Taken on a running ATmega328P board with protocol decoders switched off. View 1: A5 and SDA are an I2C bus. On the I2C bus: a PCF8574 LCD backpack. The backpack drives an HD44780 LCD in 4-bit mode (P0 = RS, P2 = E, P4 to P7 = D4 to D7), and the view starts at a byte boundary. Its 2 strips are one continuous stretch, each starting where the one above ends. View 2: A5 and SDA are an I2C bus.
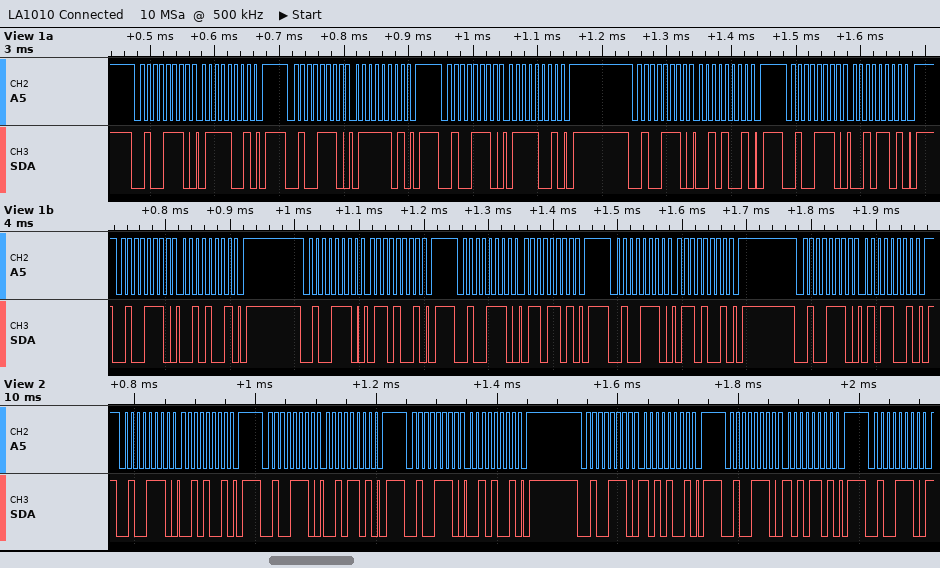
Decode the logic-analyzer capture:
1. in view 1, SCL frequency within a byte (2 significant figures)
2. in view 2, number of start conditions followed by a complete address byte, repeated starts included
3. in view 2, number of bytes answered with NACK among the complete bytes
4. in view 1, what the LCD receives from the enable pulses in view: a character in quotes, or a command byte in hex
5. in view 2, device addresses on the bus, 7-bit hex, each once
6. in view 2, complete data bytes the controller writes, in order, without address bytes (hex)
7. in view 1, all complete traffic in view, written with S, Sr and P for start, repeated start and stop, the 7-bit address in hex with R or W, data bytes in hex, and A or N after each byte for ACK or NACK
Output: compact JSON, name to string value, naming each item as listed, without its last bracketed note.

{"in view 1, SCL frequency within a byte": "100 kHz", "in view 2, number of start conditions followed by a complete address byte, repeated starts included": "6", "in view 2, number of bytes answered with NACK among the complete bytes": "0", "in view 1, what the LCD receives from the enable pulses in view: a character in quotes, or a command byte in hex": "'r'", "in view 2, device addresses on the bus, 7-bit hex, each once": "0x27", "in view 2, complete data bytes the controller writes, in order, without address bytes": "29 2D 29 A9 AD", "in view 1, all complete traffic in view, written with S, Sr and P for start, repeated start and stop, the 7-bit address in hex with R or W, data bytes in hex, and A or N after each byte for ACK or NACK": "S 27W A 79 A P S 27W A 7D A P S 27W A 79 A P S 27W A 29 A P S 27W A 2D A P S 27W A 29 A P S 27W A 69 A P S 27W A 6D A P S 27W A 69 A P S 27W A 59 A P"}
